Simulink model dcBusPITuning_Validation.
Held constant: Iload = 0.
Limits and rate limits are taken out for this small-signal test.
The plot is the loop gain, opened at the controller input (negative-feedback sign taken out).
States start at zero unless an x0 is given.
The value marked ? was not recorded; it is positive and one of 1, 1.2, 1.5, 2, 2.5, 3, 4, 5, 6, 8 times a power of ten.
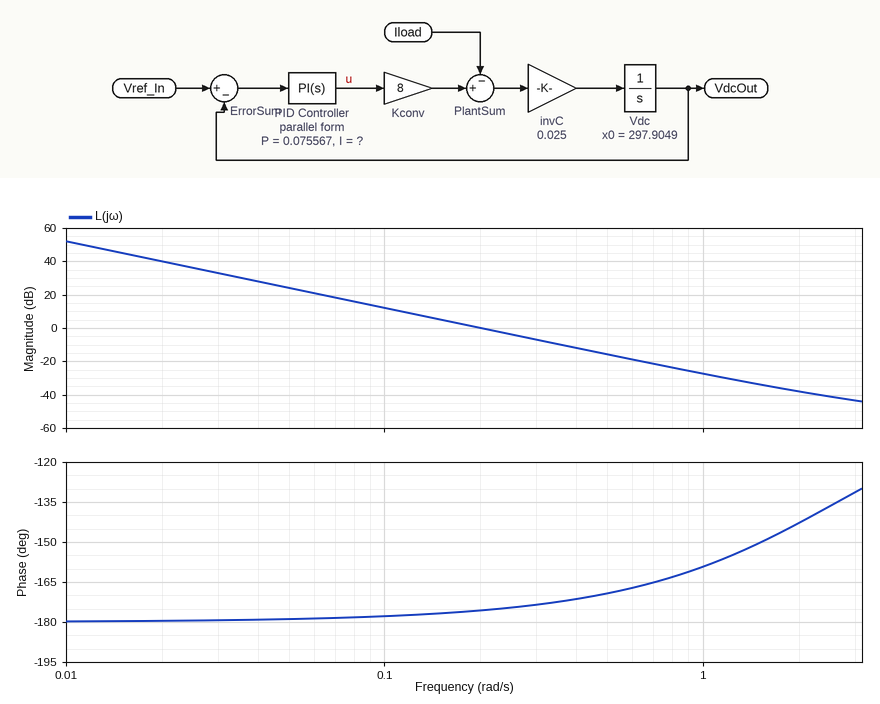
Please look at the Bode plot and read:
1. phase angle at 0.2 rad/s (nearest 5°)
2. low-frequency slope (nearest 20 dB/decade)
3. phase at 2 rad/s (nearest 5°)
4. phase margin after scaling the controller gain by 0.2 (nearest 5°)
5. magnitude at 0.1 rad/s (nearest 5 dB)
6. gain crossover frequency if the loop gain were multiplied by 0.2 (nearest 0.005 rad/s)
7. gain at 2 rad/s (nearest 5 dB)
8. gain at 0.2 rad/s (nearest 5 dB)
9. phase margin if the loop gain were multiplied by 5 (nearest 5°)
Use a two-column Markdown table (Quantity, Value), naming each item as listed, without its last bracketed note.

| Quantity | Value |
|---|---|
| phase angle at 0.2 rad/s | -175° |
| low-frequency slope | -40 dB/decade |
| phase at 2 rad/s | -145° |
| phase margin after scaling the controller gain by 0.2 | 0° |
| magnitude at 0.1 rad/s | 10 dB |
| gain crossover frequency if the loop gain were multiplied by 0.2 | 0.090 rad/s |
| gain at 2 rad/s | -40 dB |
| gain at 0.2 rad/s | 0 dB |
| phase margin if the loop gain were multiplied by 5 | 10° |
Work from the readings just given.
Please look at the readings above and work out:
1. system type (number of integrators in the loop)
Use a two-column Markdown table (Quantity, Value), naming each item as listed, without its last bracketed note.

| Quantity | Value |
|---|---|
| system type | 2 |
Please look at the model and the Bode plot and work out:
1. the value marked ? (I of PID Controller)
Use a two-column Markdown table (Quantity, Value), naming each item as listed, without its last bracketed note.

| Quantity | Value |
|---|---|
| the value marked ? | 0.2 |
